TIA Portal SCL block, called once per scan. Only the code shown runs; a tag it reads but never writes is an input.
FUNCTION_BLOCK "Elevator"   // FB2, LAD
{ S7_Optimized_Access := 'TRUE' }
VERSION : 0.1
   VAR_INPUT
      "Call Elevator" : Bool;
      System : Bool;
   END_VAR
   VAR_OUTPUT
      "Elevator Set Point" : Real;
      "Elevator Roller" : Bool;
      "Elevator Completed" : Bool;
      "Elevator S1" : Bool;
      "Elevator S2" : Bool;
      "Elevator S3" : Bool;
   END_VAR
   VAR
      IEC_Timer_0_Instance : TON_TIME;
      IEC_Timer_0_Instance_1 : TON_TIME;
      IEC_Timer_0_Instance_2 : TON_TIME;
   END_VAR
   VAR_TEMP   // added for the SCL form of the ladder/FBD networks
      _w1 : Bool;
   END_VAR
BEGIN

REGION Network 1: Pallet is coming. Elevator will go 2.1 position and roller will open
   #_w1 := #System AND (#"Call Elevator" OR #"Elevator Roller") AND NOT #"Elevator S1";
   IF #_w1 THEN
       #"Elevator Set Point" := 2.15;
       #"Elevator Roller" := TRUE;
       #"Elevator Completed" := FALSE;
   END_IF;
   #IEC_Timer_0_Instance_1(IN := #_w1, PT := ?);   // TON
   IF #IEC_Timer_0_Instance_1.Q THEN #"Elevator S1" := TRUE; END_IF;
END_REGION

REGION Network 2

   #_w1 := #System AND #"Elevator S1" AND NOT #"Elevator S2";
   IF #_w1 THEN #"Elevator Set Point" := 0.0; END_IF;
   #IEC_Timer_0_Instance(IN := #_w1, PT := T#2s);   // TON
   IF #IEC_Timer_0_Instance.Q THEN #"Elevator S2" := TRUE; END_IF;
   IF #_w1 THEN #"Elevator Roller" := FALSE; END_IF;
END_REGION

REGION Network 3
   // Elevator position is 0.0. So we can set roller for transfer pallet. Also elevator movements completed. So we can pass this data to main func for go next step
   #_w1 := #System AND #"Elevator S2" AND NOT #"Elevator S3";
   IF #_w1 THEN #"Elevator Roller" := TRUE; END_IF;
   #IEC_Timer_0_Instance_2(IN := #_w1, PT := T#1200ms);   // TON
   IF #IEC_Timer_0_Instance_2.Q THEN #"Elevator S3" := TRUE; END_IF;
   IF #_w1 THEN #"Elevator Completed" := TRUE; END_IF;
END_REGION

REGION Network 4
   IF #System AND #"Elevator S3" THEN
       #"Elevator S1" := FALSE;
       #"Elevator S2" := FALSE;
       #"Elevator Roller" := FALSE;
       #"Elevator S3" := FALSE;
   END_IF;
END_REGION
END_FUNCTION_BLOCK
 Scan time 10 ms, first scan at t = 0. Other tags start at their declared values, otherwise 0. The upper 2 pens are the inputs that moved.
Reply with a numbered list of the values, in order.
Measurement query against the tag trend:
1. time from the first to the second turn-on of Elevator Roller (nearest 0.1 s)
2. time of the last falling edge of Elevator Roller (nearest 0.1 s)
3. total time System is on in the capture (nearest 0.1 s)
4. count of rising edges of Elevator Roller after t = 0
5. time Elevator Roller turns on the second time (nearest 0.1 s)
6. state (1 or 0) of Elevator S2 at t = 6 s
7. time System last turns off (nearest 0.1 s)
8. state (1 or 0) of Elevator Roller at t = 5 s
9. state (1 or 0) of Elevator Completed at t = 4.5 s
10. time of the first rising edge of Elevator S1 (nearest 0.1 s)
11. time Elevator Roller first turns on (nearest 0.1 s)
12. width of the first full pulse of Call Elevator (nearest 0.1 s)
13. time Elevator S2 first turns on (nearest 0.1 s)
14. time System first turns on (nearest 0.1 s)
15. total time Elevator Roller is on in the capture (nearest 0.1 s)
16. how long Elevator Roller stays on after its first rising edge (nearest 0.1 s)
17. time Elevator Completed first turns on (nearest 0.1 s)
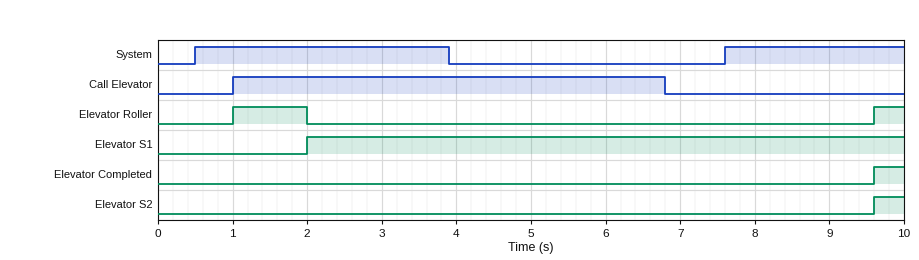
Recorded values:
1. 8.6 s
2. 2.0 s
3. 5.8 s
4. 2
5. 9.6 s
6. 0
7. 3.9 s
8. 0
9. 0
10. 2.0 s
11. 1.0 s
12. 5.8 s
13. 9.6 s
14. 0.5 s
15. 1.4 s
16. 1.0 s
17. 9.6 s
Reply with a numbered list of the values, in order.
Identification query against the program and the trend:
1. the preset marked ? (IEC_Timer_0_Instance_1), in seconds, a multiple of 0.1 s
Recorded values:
1. 1.0 s
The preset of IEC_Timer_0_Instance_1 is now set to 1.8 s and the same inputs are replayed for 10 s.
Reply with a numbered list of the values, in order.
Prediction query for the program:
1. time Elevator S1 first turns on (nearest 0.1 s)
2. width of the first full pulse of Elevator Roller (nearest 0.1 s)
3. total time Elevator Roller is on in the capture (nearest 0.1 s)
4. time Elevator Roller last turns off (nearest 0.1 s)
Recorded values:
1. 2.8 s
2. 1.8 s
3. 2.2 s
4. 2.8 s
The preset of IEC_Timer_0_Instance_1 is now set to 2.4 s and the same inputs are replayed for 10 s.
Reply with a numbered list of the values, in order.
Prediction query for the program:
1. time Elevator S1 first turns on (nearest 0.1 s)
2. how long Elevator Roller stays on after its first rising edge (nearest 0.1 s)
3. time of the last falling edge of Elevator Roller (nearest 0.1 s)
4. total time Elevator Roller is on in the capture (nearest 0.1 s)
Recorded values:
1. 3.4 s
2. 2.4 s
3. 3.4 s
4. 2.8 s
